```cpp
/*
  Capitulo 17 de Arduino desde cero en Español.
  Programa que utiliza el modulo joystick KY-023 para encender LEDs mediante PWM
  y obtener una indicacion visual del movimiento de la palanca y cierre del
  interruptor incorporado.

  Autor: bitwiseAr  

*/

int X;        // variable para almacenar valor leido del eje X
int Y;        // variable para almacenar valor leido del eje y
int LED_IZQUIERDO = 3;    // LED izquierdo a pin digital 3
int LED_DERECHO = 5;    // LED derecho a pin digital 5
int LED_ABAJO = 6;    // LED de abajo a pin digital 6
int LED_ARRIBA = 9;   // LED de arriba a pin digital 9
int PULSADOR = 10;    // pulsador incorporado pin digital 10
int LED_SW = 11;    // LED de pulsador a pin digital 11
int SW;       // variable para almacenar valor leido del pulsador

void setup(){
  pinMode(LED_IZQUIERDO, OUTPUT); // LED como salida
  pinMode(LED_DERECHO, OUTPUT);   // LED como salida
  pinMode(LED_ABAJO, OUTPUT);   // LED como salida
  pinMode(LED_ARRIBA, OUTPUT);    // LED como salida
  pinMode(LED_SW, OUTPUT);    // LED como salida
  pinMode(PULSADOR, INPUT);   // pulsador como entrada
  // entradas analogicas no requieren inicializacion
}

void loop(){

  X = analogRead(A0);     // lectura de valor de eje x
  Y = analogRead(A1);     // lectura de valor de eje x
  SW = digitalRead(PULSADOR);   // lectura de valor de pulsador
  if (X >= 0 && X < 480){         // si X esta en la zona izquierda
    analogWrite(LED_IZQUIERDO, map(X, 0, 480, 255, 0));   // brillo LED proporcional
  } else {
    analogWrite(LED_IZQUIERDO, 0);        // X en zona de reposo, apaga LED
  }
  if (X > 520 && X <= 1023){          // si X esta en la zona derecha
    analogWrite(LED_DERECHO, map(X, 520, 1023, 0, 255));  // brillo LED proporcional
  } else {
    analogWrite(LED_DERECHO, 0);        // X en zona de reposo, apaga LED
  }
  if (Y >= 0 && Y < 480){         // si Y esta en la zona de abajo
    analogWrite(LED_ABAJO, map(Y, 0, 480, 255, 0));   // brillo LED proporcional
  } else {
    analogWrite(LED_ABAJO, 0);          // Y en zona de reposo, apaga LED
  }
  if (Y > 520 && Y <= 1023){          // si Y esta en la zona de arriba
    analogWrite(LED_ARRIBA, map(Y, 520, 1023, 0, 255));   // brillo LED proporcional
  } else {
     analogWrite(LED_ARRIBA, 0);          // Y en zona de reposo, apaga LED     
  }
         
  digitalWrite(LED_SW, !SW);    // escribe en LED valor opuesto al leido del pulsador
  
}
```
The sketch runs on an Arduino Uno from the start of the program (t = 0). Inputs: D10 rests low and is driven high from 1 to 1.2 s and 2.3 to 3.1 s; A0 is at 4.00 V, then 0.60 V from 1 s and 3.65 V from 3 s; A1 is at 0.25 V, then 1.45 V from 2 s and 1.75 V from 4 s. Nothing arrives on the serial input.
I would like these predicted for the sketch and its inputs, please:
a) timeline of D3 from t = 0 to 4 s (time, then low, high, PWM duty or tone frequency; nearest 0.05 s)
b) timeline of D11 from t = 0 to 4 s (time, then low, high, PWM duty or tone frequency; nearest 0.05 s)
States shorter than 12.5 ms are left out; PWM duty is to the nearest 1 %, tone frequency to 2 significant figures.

0 s low; 1 s PWM 75 %; 3 s low
0 s high; 1 s low; 1.2 s high; 2.3 s low; 3.1 s high
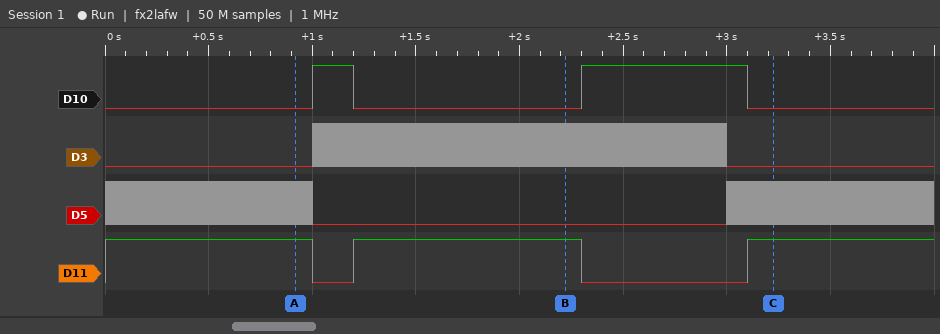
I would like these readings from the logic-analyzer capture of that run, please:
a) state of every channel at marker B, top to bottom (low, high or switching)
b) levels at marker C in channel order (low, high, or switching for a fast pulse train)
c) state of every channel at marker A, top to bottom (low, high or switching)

D10 low, D3 switching, D5 low, D11 high
D10 low, D3 low, D5 switching, D11 high
D10 low, D3 low, D5 switching, D11 high
